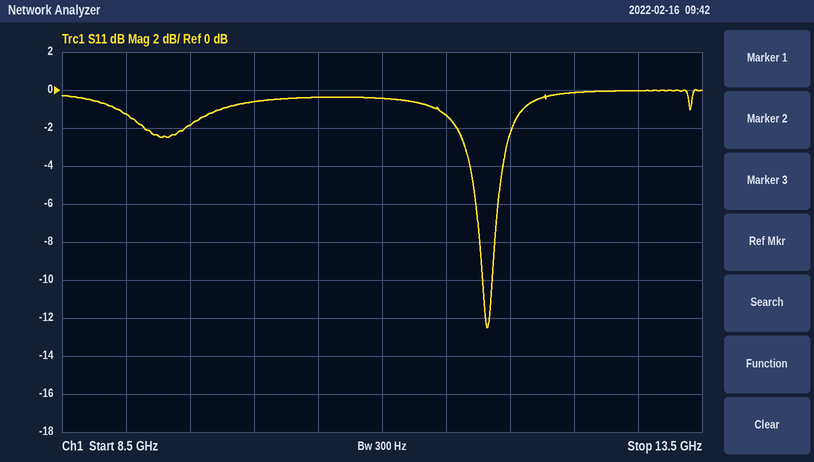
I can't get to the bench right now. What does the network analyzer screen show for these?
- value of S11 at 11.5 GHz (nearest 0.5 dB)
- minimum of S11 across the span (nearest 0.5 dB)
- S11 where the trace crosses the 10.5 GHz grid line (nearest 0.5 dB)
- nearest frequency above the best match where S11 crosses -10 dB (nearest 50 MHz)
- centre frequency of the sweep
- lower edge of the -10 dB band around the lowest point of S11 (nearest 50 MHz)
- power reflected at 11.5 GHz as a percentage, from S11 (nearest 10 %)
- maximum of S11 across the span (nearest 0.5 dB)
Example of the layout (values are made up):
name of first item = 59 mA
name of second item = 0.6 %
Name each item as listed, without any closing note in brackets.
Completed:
value of S11 at 11.5 GHz = -1.5 dB
minimum of S11 across the span = -12.5 dB
S11 where the trace crosses the 10.5 GHz grid line = -0.5 dB
nearest frequency above the best match where S11 crosses -10 dB = 11.85 GHz
centre frequency of the sweep = 11 GHz
lower edge of the -10 dB band around the lowest point of S11 = 11.80 GHz
power reflected at 11.5 GHz as a percentage, from S11 = 70 %
maximum of S11 across the span = 0.0 dB
